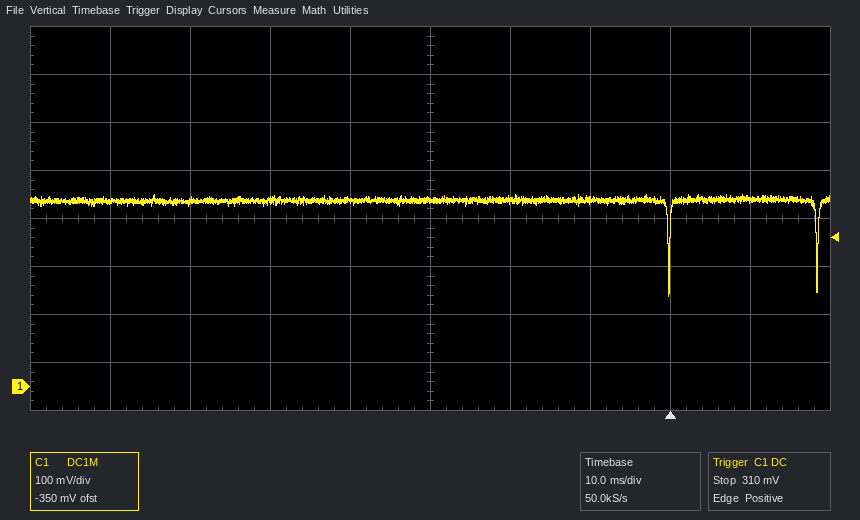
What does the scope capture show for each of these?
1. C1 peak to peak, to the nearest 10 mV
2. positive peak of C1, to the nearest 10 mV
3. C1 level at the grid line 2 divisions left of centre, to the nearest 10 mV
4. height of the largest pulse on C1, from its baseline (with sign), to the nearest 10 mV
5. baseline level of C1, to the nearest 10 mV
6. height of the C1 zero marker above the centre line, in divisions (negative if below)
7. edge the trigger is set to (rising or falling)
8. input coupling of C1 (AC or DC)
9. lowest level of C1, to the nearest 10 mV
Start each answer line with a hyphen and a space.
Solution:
- 210 mV
- 400 mV
- 390 mV
- -200 mV
- 390 mV
- -3.5 div
- rising
- DC
- 190 mV
